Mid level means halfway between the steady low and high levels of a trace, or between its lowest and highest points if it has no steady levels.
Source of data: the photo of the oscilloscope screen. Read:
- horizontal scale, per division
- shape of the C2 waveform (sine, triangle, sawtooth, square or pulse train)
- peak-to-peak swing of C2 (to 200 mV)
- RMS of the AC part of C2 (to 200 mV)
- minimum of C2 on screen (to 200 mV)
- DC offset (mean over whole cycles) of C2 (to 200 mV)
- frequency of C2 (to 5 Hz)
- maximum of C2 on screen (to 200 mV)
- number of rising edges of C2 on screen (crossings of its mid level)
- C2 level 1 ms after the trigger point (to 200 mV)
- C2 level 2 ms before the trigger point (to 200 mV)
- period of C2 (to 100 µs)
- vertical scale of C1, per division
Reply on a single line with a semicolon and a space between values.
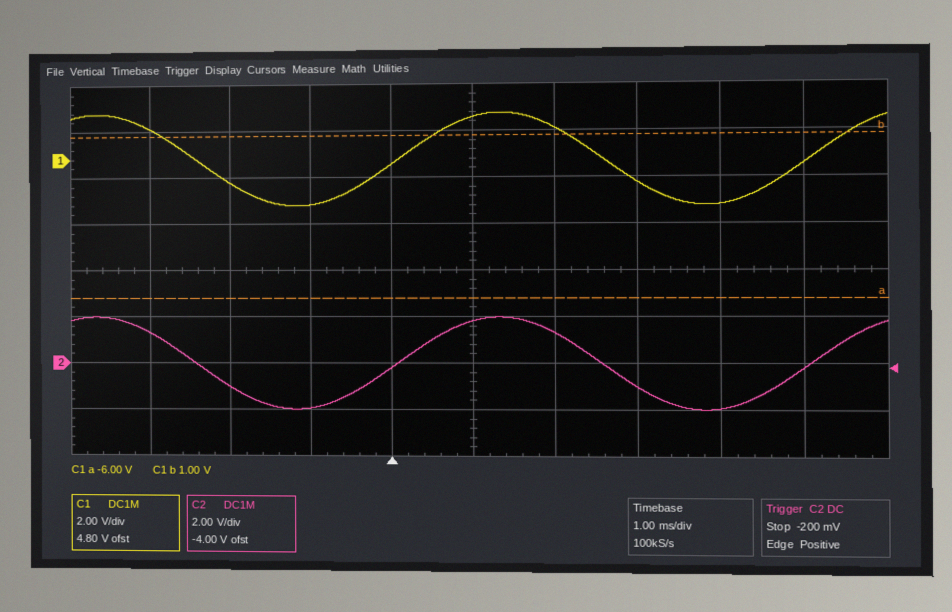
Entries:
1 ms; sine; 4.0 V; 1.4 V; -2.0 V; 0.0 V; 200 Hz; 2.0 V; 2; 1.8 V; -1.0 V; 5.0 ms; 2 V
